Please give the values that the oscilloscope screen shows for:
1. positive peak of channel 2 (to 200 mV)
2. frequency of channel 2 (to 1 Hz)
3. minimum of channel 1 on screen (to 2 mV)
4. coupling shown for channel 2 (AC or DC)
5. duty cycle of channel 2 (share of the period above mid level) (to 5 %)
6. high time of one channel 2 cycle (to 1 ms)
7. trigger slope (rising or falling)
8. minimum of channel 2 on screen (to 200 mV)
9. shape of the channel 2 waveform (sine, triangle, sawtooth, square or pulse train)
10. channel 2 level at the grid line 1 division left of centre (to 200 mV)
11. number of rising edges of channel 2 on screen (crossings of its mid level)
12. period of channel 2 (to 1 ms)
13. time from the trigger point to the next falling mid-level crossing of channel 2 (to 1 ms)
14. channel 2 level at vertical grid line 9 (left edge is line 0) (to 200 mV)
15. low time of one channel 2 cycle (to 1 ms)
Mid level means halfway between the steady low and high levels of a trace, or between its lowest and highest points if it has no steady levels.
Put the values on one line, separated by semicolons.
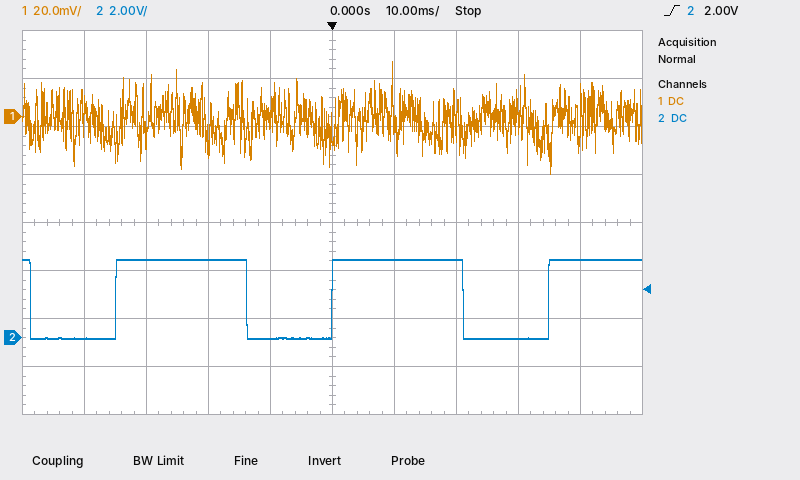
3.2 V; 29 Hz; -24 mV; DC; 60 %; 21 ms; rising; 0.0 V; pulse train; 0.0 V; 3; 35 ms; 21 ms; 3.2 V; 14 ms
